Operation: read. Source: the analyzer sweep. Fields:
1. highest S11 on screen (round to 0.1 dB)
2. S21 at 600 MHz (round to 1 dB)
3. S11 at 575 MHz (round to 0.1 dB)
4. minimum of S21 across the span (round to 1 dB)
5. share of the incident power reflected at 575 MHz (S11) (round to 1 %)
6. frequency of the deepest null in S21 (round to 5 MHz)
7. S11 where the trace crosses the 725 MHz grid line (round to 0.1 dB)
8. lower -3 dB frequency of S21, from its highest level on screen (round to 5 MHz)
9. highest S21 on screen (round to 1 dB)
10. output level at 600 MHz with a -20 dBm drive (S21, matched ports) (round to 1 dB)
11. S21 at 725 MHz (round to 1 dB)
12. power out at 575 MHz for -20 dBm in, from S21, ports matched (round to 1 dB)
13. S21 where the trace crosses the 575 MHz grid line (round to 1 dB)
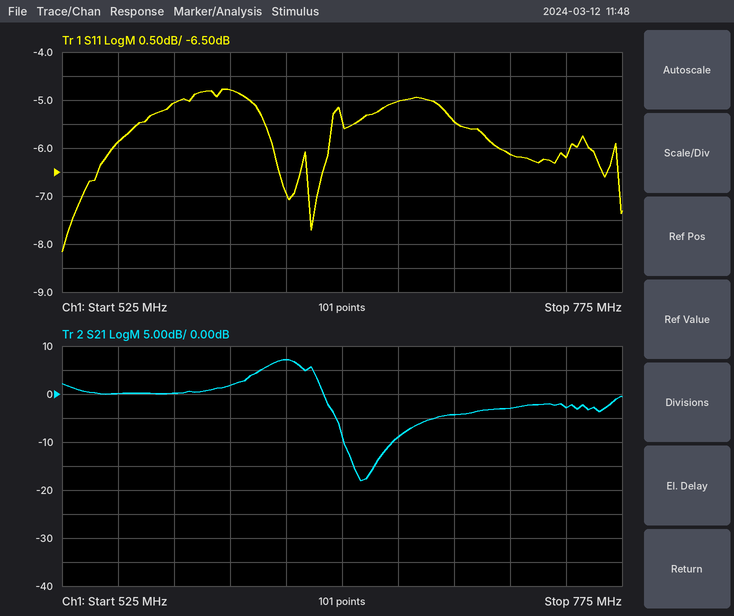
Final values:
-4.8 dB
2 dB
-5.1 dB
-18 dB
31 %
660 MHz
-6.1 dB
610 MHz
7 dB
-18 dBm
-3 dB
-20 dBm
0 dB
